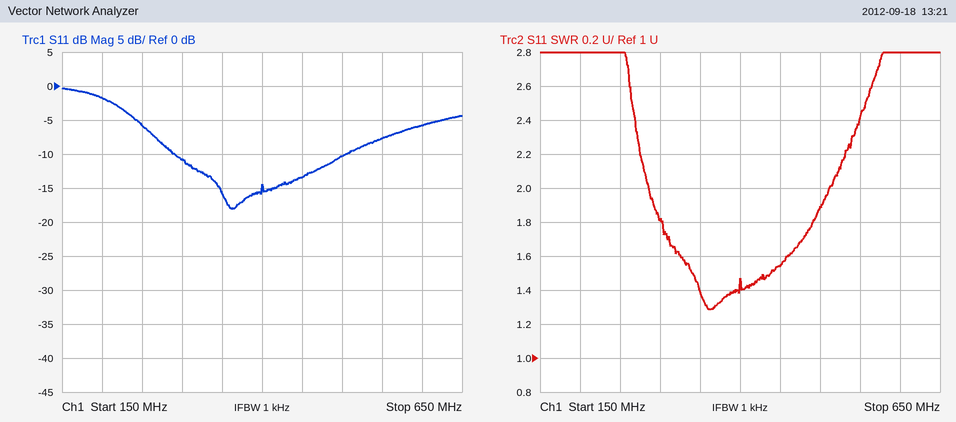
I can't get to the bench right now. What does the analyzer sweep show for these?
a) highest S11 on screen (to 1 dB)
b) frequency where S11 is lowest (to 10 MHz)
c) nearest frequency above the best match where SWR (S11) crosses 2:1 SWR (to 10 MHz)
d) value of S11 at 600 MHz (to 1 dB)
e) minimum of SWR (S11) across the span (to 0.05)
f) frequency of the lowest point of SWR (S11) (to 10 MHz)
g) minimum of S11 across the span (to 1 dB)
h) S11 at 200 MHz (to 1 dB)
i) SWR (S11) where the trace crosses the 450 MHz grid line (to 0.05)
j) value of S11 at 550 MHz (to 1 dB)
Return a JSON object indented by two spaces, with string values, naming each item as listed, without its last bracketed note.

{
  "highest S11 on screen": "0 dB",
  "frequency where S11 is lowest": "360 MHz",
  "nearest frequency above the best match where SWR (S11) crosses 2:1 SWR": "510 MHz",
  "value of S11 at 600 MHz": "-6 dB",
  "minimum of SWR (S11) across the span": "1.30",
  "frequency of the lowest point of SWR (S11)": "360 MHz",
  "minimum of S11 across the span": "-18 dB",
  "S11 at 200 MHz": "-2 dB",
  "SWR (S11) where the trace crosses the 450 MHz grid line": "1.55",
  "value of S11 at 550 MHz": "-8 dB"
}
